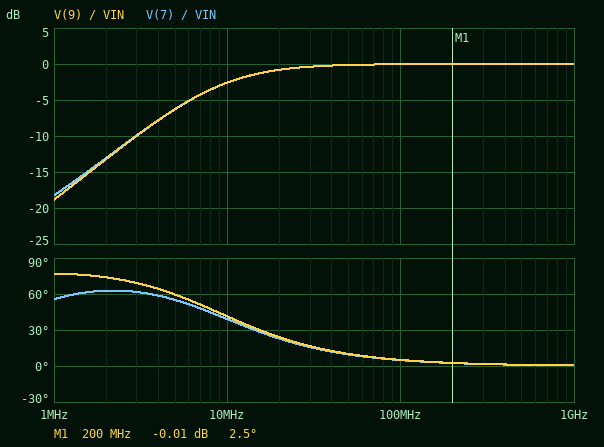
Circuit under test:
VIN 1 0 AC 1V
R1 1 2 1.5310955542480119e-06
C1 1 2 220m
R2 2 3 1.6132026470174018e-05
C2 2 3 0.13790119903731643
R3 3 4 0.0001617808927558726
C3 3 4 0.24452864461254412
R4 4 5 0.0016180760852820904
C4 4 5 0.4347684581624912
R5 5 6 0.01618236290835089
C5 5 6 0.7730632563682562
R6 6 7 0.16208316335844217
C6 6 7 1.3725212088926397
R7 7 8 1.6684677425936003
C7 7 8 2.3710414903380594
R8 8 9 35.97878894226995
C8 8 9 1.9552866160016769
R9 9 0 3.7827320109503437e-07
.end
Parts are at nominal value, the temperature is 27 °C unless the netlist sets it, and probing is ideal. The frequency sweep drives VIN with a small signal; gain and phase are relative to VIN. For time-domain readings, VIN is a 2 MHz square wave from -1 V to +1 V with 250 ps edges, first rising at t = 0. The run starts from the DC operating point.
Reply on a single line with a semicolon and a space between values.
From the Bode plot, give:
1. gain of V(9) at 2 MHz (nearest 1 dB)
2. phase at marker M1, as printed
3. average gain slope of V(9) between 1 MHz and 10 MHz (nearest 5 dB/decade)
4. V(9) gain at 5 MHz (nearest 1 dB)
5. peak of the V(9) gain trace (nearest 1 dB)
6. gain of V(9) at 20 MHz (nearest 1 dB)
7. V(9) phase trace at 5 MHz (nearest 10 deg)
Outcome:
-13 dB; 2.5 deg; 15 dB/decade; -6 dB; 0 dB; -1 dB; 60 deg
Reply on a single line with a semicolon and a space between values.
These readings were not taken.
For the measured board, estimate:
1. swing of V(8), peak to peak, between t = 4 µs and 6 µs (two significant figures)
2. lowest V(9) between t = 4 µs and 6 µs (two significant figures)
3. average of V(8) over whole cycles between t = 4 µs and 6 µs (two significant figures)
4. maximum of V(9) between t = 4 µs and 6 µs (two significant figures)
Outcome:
3.9 V; -2.0 V; -900 mV; 2.0 V
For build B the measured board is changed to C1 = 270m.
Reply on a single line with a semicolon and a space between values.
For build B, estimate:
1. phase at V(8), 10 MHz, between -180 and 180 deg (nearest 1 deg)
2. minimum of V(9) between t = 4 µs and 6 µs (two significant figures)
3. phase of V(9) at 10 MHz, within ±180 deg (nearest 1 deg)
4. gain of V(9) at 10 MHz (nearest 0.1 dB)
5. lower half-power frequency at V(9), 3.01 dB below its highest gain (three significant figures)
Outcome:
39 deg; -2.0 V; 40 deg; -2.4 dB; 8.63 MHz
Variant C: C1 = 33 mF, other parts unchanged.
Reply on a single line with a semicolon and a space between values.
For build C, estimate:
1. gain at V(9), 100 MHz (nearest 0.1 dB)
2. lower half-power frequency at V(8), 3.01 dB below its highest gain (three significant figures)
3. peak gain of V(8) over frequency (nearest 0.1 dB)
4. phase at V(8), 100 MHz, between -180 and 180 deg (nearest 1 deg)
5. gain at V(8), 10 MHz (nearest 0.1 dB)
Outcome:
-0.2 dB; 21.5 MHz; 0 dB; 11 deg; -7.3 dB
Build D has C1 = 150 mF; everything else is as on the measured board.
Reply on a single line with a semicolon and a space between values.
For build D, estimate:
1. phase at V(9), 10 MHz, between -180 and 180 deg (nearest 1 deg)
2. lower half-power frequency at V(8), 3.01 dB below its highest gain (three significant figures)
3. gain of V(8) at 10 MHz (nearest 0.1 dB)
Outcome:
44 deg; 9.99 MHz; -3.0 dB
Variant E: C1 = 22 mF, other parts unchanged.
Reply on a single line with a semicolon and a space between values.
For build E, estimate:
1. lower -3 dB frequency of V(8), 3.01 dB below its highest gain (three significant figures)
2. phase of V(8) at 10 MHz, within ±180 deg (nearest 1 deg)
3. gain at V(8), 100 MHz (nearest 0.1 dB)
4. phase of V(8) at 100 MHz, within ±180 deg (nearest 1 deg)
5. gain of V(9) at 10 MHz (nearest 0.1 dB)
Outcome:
29.0 MHz; 51 deg; -0.4 dB; 14 deg; -9.1 dB
